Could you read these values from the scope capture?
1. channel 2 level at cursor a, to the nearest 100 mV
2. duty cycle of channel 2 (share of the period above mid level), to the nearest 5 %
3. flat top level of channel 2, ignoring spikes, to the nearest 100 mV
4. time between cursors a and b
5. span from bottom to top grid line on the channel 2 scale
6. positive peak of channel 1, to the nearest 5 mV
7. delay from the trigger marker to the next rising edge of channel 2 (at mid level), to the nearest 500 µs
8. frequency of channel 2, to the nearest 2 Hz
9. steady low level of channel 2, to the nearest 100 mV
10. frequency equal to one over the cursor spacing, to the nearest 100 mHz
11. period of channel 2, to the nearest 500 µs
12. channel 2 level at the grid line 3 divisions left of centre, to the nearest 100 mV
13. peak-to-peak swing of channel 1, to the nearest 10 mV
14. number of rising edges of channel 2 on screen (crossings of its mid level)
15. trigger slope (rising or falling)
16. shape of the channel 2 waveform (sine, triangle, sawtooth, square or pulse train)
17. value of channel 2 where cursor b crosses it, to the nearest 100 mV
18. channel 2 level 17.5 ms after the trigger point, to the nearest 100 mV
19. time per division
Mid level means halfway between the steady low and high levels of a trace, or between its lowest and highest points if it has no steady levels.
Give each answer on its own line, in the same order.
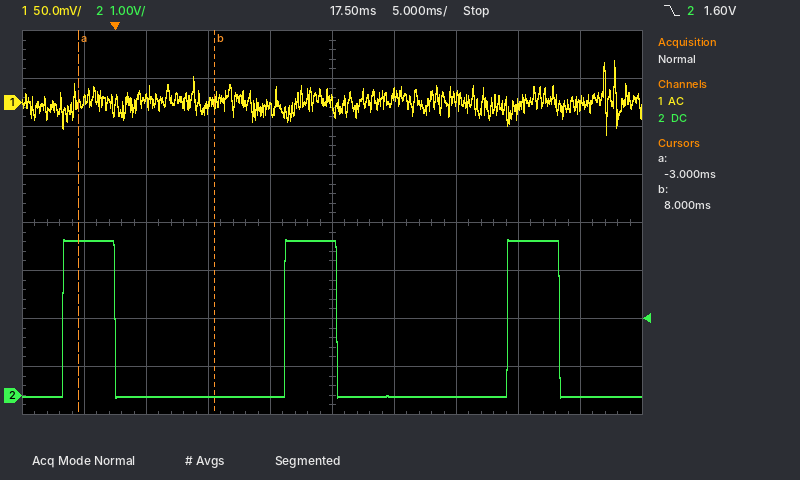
3.2 V
25 %
3.2 V
11.0 ms
8 V
45 mV
13.5 ms
56 Hz
0.0 V
90.9 Hz
18.0 ms
0.0 V
80 mV
3
falling
pulse train
0.0 V
3.2 V
5 ms
